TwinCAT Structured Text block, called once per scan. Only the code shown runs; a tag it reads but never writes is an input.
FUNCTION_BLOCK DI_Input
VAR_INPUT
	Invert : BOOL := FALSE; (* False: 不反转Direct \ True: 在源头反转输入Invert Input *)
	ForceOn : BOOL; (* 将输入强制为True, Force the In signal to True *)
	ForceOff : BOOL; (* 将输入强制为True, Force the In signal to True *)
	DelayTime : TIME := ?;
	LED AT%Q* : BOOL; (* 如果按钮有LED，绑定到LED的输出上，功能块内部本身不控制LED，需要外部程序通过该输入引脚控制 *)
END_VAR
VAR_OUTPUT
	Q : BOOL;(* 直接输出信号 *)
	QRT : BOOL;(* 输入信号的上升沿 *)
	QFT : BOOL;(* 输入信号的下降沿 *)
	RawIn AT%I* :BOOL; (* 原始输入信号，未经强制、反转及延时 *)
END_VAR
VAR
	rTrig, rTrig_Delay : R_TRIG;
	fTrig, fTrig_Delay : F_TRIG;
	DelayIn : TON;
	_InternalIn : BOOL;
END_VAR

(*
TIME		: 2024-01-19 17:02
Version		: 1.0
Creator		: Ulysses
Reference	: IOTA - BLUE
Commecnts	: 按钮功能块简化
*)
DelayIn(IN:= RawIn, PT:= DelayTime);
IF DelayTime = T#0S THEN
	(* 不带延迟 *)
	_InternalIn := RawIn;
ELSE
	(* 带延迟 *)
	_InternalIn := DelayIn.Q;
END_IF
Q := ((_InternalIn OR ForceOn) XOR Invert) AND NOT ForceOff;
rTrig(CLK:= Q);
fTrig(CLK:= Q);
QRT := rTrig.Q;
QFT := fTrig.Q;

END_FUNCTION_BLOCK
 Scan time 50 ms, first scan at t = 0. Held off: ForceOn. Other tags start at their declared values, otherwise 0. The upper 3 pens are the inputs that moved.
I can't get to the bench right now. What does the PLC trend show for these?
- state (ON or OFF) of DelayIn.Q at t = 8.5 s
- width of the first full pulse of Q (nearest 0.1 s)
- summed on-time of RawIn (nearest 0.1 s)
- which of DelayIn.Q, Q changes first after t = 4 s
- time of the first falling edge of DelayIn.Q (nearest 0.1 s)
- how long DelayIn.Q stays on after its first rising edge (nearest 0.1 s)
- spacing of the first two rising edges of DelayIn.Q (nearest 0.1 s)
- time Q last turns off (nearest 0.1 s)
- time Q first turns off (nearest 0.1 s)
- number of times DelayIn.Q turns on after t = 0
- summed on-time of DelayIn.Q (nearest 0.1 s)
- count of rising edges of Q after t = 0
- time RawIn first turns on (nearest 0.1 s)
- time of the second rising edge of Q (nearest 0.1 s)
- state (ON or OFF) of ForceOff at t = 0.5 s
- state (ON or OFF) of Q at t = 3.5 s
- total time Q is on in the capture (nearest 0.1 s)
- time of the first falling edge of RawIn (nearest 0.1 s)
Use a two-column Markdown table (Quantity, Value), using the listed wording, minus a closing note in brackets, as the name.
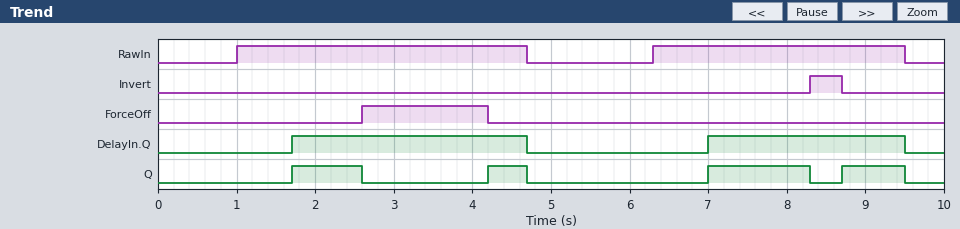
| Quantity | Value |
|---|---|
| state (ON or OFF) of DelayIn.Q at t = 8.5 s | ON |
| width of the first full pulse of Q | 0.9 s |
| summed on-time of RawIn | 6.9 s |
| which of DelayIn.Q, Q changes first after t = 4 s | Q |
| time of the first falling edge of DelayIn.Q | 4.7 s |
| how long DelayIn.Q stays on after its first rising edge | 3.0 s |
| spacing of the first two rising edges of DelayIn.Q | 5.3 s |
| time Q last turns off | 9.5 s |
| time Q first turns off | 2.6 s |
| number of times DelayIn.Q turns on after t = 0 | 2 |
| summed on-time of DelayIn.Q | 5.5 s |
| count of rising edges of Q after t = 0 | 4 |
| time RawIn first turns on | 1.0 s |
| time of the second rising edge of Q | 4.2 s |
| state (ON or OFF) of ForceOff at t = 0.5 s | OFF |
| state (ON or OFF) of Q at t = 3.5 s | OFF |
| total time Q is on in the capture | 3.5 s |
| time of the first falling edge of RawIn | 4.7 s |
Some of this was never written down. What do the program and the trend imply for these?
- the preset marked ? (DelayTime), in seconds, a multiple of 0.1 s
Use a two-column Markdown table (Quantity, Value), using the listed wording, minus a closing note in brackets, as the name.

| Quantity | Value |
|---|---|
| the preset marked ? (DelayTime), in seconds, a multiple of 0.1 s | 0.7 s |
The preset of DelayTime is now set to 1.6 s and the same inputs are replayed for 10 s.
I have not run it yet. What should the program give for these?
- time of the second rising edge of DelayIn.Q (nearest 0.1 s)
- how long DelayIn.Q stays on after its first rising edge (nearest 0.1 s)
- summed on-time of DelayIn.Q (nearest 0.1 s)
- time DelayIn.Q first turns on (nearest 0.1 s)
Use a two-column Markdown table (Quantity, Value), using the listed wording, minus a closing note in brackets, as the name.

| Quantity | Value |
|---|---|
| time of the second rising edge of DelayIn.Q | 7.9 s |
| how long DelayIn.Q stays on after its first rising edge | 2.1 s |
| summed on-time of DelayIn.Q | 3.7 s |
| time DelayIn.Q first turns on | 2.6 s |
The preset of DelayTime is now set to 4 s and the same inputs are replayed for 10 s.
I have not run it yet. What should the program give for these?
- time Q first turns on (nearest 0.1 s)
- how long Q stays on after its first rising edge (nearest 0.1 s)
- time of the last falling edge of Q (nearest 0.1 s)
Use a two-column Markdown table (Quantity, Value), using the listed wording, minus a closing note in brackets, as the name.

| Quantity | Value |
|---|---|
| time Q first turns on | 8.3 s |
| how long Q stays on after its first rising edge | 0.4 s |
| time of the last falling edge of Q | 8.7 s |
